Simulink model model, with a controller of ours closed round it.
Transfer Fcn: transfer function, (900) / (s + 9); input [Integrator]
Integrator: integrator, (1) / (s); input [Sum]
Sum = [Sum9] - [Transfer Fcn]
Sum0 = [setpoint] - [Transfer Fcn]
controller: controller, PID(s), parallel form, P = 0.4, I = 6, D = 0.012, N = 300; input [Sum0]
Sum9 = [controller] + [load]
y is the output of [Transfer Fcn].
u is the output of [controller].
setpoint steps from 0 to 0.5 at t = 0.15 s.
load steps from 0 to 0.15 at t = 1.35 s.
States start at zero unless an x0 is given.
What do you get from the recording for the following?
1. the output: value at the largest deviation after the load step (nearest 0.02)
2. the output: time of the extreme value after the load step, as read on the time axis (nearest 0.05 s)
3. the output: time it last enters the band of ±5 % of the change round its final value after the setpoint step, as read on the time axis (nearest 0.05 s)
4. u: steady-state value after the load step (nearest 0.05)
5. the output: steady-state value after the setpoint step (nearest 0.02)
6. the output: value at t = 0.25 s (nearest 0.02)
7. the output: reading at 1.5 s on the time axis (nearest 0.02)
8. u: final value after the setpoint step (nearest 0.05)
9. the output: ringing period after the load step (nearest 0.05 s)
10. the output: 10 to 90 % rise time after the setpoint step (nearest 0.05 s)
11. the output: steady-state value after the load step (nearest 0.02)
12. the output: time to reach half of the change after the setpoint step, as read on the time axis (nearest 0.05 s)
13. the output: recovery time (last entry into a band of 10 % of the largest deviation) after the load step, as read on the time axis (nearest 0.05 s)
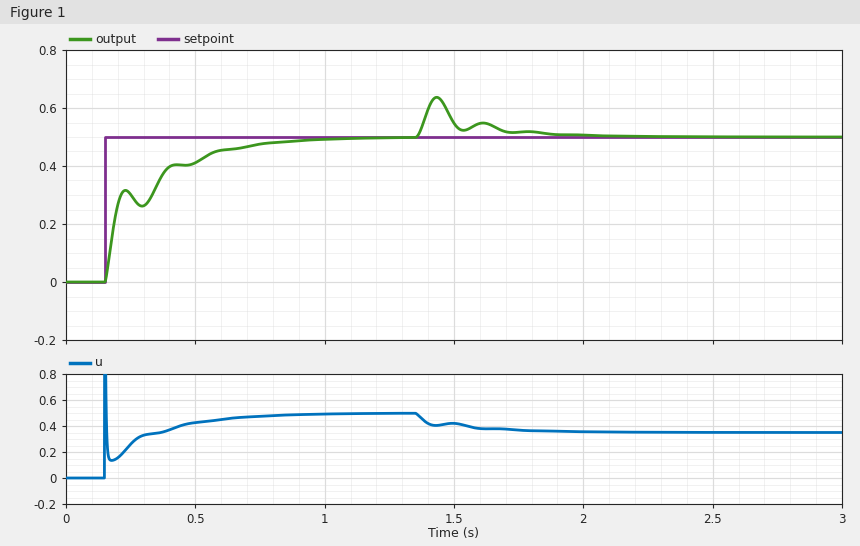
0.64
1.45 s
0.75 s
0.35
0.50
0.30
0.54
0.50
0.20 s
0.40 s
0.50
0.20 s
1.85 s
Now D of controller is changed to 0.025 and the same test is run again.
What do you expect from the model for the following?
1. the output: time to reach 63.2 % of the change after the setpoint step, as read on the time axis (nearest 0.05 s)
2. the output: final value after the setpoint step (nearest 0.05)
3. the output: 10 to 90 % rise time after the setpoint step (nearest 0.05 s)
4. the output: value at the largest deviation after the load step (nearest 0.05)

0.35 s
0.50
0.45 s
0.60
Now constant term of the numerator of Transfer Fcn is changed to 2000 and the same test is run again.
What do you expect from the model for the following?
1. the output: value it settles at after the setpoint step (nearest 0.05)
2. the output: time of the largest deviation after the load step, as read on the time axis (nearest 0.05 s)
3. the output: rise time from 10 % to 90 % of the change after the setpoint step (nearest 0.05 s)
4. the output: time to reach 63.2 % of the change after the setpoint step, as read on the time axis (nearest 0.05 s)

0.50
1.40 s
0.45 s
0.30 s
